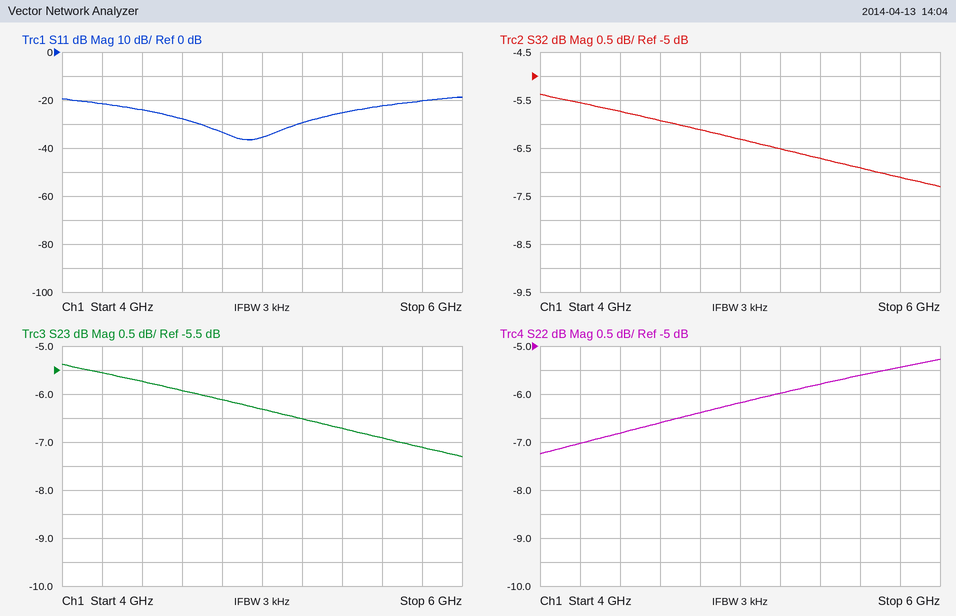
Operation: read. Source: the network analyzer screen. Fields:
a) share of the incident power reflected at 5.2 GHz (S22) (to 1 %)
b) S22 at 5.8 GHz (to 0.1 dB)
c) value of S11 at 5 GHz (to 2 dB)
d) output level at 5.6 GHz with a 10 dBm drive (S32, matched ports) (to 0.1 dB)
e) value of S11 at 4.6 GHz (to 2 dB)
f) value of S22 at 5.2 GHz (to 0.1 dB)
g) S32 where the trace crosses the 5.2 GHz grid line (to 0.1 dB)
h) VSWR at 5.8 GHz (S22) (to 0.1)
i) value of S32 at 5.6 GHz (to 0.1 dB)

25 %
-5.4 dB
-36 dB
3.1 dBm
-28 dB
-6.0 dB
-6.5 dB
3.3
-6.9 dB
